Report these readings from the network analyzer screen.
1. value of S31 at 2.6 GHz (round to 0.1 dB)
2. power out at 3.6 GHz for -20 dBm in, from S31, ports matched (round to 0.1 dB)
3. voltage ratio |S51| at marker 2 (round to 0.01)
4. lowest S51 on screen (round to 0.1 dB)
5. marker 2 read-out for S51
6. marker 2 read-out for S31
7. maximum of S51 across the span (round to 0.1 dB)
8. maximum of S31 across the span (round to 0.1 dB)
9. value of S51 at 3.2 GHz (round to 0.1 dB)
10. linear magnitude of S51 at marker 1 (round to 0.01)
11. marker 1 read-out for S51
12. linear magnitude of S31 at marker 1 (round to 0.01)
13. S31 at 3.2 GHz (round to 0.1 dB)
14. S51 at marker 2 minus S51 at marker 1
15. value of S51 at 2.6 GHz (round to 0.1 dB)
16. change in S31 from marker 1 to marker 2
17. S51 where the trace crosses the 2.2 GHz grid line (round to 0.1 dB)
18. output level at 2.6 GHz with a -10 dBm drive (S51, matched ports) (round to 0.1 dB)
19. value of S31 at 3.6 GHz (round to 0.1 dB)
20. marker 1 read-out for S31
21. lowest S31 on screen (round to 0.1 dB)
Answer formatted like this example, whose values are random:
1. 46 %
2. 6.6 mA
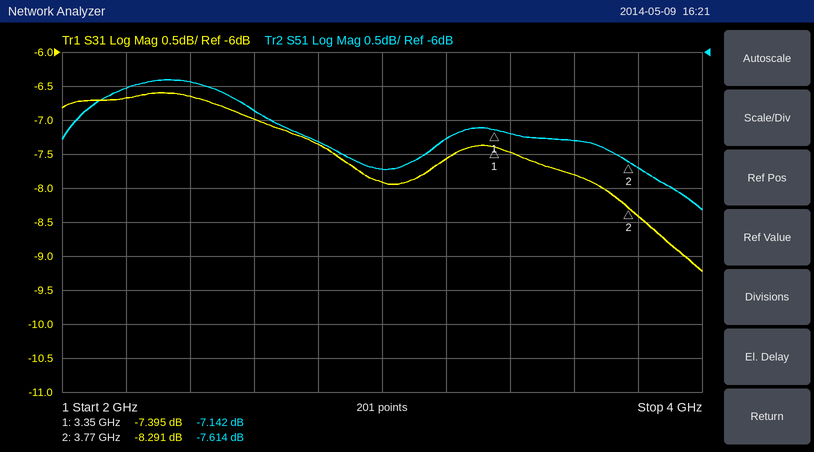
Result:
1. -7.0 dB
2. -27.8 dBm
3. 0.42
4. -8.3 dB
5. -7.614 dB
6. -8.291 dB
7. -6.4 dB
8. -6.6 dB
9. -7.3 dB
10. 0.44
11. -7.142 dB
12. 0.43
13. -7.6 dB
14. -0.472 dB
15. -6.9 dB
16. -0.896 dB
17. -6.5 dB
18. -16.9 dBm
19. -7.8 dB
20. -7.395 dB
21. -9.2 dB
